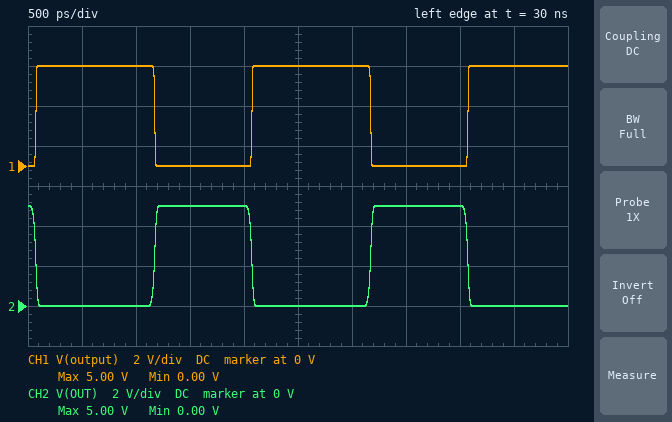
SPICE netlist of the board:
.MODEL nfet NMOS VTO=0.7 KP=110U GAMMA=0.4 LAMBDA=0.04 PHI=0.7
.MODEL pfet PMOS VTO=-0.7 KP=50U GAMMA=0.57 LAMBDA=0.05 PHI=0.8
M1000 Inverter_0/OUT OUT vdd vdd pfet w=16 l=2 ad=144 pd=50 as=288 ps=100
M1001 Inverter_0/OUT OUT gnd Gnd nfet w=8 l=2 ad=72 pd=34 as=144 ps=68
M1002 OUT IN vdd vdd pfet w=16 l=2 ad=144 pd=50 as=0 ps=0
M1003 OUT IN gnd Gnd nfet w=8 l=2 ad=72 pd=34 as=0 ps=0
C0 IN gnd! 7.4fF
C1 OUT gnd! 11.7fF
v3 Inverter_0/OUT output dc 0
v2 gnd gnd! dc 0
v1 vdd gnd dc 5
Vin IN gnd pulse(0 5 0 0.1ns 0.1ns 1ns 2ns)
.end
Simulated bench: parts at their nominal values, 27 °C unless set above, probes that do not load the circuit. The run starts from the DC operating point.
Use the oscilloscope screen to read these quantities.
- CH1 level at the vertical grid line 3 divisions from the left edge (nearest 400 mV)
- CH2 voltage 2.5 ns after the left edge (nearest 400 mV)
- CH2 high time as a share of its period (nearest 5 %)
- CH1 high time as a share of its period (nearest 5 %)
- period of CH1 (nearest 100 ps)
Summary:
0 V
0 V
45 %
55 %
2.0 ns
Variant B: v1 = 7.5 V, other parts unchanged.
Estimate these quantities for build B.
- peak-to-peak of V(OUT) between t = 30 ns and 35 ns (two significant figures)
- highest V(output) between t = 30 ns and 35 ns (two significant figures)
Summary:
7.0 V
7.5 V
